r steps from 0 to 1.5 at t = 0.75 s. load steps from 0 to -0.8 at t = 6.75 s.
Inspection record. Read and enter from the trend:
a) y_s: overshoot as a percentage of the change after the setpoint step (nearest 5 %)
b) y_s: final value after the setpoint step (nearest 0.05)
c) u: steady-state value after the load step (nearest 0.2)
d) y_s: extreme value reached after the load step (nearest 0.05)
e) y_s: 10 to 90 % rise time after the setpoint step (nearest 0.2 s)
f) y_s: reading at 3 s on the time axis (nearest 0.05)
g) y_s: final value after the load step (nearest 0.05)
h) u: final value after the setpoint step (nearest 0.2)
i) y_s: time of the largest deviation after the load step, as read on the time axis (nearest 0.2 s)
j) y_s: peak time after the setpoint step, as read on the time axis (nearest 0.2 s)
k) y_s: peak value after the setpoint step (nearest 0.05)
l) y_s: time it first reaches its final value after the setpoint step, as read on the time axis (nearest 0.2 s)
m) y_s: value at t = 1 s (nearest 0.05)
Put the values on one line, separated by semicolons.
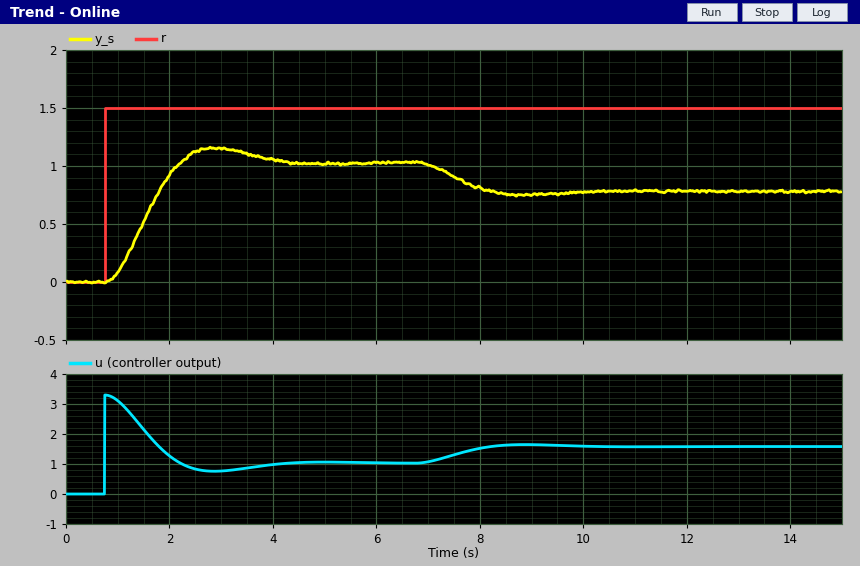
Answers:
10 %; 1.05; 1.6; 0.75; 1.0 s; 1.15; 0.80; 1.0; 8.8 s; 2.8 s; 1.15; 2.2 s; 0.10
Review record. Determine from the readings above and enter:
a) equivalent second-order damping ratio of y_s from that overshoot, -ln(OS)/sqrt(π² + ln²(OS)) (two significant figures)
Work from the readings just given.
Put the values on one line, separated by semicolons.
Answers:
0.59
